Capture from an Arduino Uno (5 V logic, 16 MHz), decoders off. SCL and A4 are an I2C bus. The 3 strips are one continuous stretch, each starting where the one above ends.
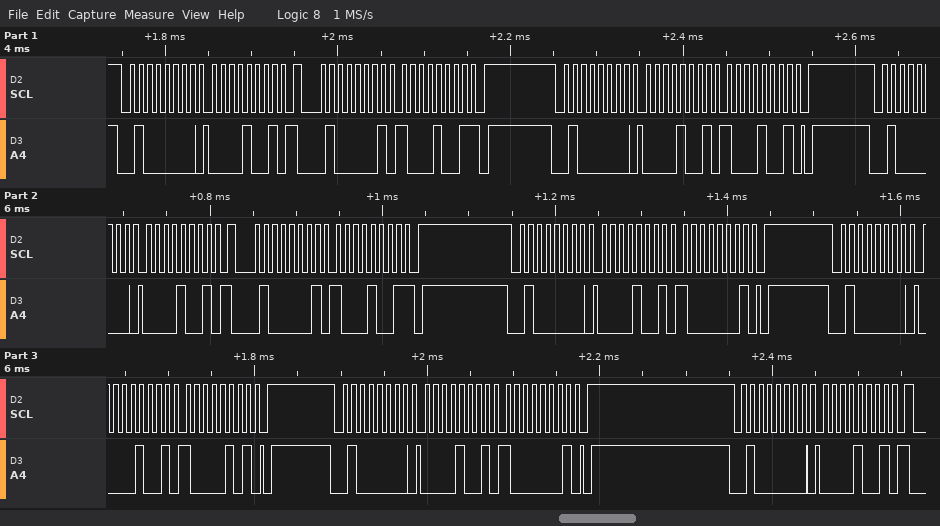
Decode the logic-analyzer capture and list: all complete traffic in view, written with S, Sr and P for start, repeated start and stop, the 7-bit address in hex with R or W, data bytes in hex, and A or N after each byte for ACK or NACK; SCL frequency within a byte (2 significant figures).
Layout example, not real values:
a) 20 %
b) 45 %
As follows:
a) S 20W A 09 A Sr 20R A 89 N P S 20W A 09 A 89 A P S 20W A 09 A Sr 20R A 89 N P S 20W A 09 A 81 A P S 20W A 09 A 85 A P S 20W A 09 A 81 A P S 20W A 09 A
b) 100 kHz
